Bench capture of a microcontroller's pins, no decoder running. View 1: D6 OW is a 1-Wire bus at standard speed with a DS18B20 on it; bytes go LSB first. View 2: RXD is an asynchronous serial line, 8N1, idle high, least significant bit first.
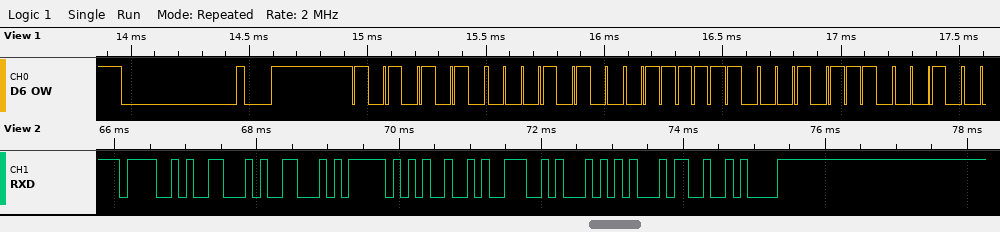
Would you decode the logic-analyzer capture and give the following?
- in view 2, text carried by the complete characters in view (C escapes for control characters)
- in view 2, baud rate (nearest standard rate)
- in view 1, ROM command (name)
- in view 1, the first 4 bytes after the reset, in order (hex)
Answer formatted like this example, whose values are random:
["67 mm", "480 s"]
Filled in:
["\"OFF_INT4\\n\"", "9600 baud", "Match ROM", "55 28 7E 74"]
